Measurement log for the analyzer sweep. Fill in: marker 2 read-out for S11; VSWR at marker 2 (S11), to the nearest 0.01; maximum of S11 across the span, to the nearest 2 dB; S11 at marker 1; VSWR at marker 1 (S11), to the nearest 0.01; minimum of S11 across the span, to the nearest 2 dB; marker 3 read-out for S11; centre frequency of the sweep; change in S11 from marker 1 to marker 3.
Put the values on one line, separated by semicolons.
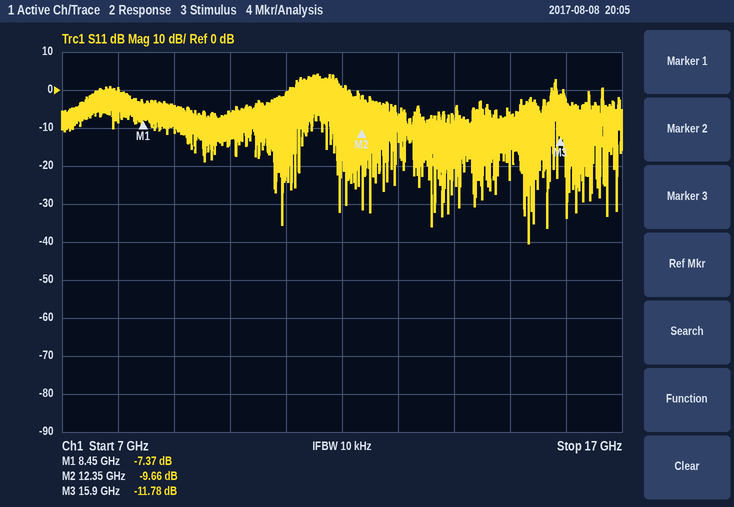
-9.66 dB; 1.98; 4 dB; -7.37 dB; 2.50; -40 dB; -11.78 dB; 12 GHz; -4.41 dB
